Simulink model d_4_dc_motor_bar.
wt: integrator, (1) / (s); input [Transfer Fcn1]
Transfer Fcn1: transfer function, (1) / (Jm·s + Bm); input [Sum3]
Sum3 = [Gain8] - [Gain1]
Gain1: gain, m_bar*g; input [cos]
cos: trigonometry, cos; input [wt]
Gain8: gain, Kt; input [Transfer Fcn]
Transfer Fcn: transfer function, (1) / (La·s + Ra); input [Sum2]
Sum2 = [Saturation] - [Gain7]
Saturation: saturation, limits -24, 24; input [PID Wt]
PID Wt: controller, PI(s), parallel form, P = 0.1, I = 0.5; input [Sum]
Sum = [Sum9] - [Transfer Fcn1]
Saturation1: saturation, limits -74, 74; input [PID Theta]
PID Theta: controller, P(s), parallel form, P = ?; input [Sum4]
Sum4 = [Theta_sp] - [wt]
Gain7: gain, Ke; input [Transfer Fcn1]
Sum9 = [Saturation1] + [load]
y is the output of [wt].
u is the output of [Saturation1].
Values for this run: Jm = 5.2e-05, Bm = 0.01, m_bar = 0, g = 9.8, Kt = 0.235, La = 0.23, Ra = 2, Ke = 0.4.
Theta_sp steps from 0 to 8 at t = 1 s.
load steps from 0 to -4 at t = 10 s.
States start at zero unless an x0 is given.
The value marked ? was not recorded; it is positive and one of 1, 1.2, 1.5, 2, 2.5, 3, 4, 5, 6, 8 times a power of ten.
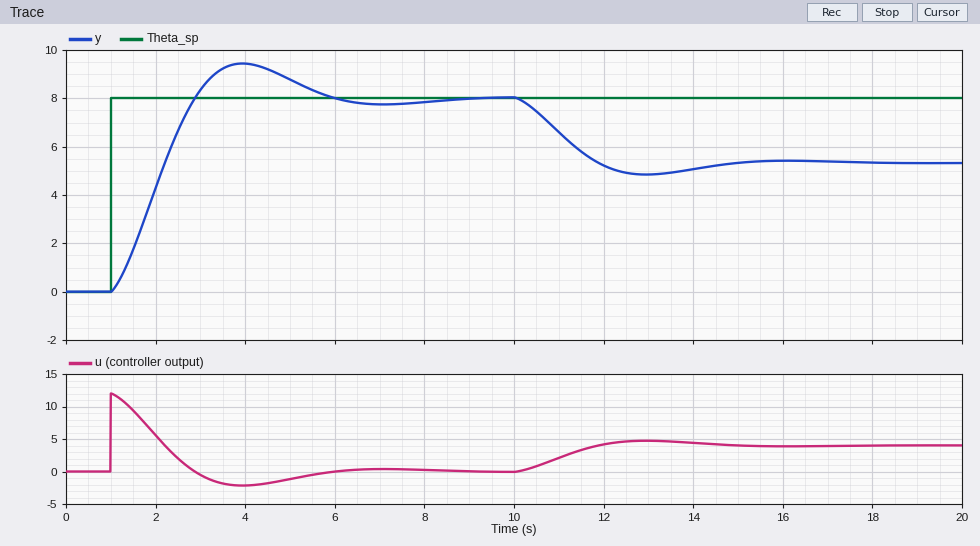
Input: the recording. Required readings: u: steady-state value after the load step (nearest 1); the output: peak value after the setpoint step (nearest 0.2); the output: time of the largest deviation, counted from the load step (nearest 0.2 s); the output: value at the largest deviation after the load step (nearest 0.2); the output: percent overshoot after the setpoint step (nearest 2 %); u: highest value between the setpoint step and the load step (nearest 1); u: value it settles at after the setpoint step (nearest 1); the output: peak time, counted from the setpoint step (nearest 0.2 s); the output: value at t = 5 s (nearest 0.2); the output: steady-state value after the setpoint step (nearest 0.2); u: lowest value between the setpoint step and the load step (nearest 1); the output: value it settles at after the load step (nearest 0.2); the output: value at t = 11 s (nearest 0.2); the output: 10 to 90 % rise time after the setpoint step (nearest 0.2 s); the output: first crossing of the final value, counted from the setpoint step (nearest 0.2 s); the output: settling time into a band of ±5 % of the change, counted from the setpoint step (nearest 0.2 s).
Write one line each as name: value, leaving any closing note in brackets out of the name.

u: steady-state value after the load step: 4
the output: peak value after the setpoint step: 9.4
the output: time of the largest deviation, counted from the load step: 3.0 s
the output: value at the largest deviation after the load step: 4.8
the output: percent overshoot after the setpoint step: 18 %
u: highest value between the setpoint step and the load step: 12
u: value it settles at after the setpoint step: 0
the output: peak time, counted from the setpoint step: 3.0 s
the output: value at t = 5 s: 8.8
the output: steady-state value after the setpoint step: 8.0
u: lowest value between the setpoint step and the load step: -2
the output: value it settles at after the load step: 5.4
the output: value at t = 11 s: 6.6
the output: 10 to 90 % rise time after the setpoint step: 1.4 s
the output: first crossing of the final value, counted from the setpoint step: 1.8 s
the output: settling time into a band of ±5 % of the change, counted from the setpoint step: 4.4 s
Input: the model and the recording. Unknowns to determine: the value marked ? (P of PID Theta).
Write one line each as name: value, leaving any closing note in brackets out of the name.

the value marked ?: 1.5
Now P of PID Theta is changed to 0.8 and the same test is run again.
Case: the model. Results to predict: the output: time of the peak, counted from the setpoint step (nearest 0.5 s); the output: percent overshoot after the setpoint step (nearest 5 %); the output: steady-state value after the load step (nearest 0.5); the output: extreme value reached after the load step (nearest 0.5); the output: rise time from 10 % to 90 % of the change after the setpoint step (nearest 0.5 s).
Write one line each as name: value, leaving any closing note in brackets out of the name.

the output: time of the peak, counted from the setpoint step: 4.5 s
the output: percent overshoot after the setpoint step: 10 %
the output: steady-state value after the load step: 3.0
the output: extreme value reached after the load step: 2.5
the output: rise time from 10 % to 90 % of the change after the setpoint step: 2.0 s
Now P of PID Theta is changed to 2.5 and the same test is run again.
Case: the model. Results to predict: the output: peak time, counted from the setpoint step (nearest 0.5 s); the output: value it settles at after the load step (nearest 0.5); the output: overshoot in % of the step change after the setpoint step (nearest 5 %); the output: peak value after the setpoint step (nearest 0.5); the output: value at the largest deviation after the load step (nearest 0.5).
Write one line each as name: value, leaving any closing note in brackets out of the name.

the output: peak time, counted from the setpoint step: 2.0 s
the output: value it settles at after the load step: 6.5
the output: overshoot in % of the step change after the setpoint step: 25 %
the output: peak value after the setpoint step: 10.0
the output: value at the largest deviation after the load step: 6.0
